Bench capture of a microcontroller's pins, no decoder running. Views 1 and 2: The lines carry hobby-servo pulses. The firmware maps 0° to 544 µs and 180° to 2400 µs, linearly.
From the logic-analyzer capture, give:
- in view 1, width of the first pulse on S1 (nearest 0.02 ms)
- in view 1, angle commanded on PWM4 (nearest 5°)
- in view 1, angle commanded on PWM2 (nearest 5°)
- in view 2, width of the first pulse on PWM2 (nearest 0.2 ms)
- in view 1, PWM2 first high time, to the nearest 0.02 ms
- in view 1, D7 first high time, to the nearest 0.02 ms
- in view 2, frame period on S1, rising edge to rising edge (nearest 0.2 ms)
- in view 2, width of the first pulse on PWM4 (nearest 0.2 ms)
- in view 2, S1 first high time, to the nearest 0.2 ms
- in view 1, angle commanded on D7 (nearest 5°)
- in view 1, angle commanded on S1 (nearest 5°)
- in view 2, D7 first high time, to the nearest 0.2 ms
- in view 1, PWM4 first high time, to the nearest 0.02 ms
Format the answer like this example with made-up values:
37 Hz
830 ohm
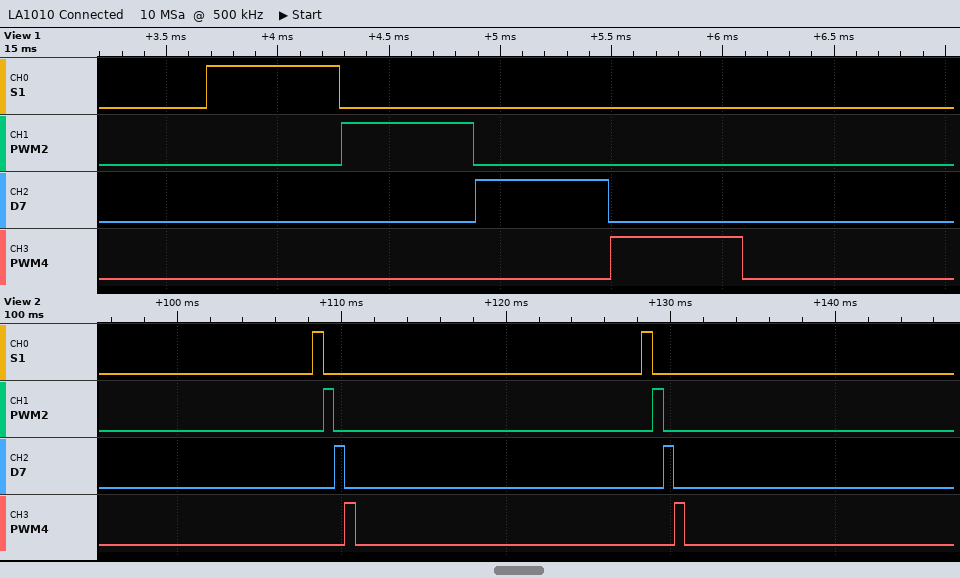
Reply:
0.60 ms
5°
5°
0.6 ms
0.60 ms
0.60 ms
20.0 ms
0.6 ms
0.6 ms
5°
5°
0.6 ms
0.60 ms
